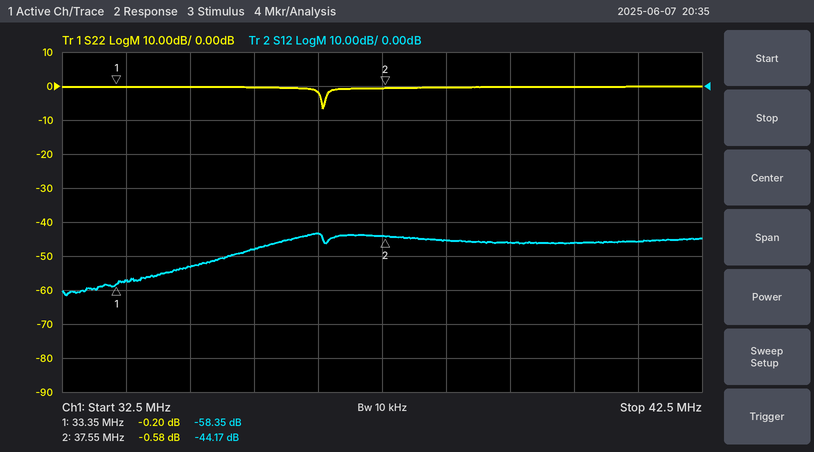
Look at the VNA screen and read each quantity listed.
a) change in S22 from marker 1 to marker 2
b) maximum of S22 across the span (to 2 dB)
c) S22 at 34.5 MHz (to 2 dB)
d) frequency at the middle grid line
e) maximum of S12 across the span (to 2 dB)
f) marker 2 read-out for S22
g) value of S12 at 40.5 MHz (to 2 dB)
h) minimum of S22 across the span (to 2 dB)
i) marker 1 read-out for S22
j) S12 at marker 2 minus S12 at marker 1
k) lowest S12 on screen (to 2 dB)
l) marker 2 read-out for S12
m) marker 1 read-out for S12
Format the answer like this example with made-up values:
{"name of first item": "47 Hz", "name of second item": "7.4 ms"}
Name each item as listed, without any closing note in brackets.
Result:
{"change in S22 from marker 1 to marker 2": "-0.38 dB", "maximum of S22 across the span": "0 dB", "S22 at 34.5 MHz": "0 dB", "frequency at the middle grid line": "37.5 MHz", "maximum of S12 across the span": "-44 dB", "marker 2 read-out for S22": "-0.58 dB", "value of S12 at 40.5 MHz": "-46 dB", "minimum of S22 across the span": "-6 dB", "marker 1 read-out for S22": "-0.20 dB", "S12 at marker 2 minus S12 at marker 1": "14.18 dB", "lowest S12 on screen": "-62 dB", "marker 2 read-out for S12": "-44.17 dB", "marker 1 read-out for S12": "-58.35 dB"}
